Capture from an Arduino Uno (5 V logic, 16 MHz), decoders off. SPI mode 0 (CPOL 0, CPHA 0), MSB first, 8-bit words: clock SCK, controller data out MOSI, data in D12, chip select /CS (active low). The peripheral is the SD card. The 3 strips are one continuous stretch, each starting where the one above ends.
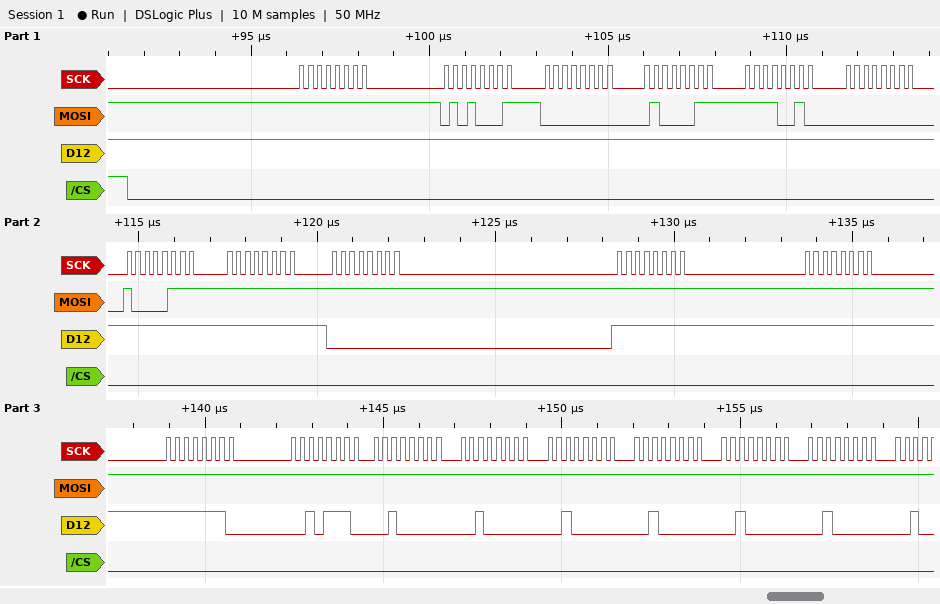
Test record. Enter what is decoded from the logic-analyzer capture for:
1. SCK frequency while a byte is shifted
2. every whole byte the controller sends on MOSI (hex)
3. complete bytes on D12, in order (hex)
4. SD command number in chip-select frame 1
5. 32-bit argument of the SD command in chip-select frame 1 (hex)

4 MHz
FF 51 00 43 F2 00 87 FF FF FF FF FF FF FF FF FF FF FF FF
FF FF FF FF FF FF FF FF 00 FF FF FE 2E 20 20 20 20 20 20
CMD17
0x0043F200
